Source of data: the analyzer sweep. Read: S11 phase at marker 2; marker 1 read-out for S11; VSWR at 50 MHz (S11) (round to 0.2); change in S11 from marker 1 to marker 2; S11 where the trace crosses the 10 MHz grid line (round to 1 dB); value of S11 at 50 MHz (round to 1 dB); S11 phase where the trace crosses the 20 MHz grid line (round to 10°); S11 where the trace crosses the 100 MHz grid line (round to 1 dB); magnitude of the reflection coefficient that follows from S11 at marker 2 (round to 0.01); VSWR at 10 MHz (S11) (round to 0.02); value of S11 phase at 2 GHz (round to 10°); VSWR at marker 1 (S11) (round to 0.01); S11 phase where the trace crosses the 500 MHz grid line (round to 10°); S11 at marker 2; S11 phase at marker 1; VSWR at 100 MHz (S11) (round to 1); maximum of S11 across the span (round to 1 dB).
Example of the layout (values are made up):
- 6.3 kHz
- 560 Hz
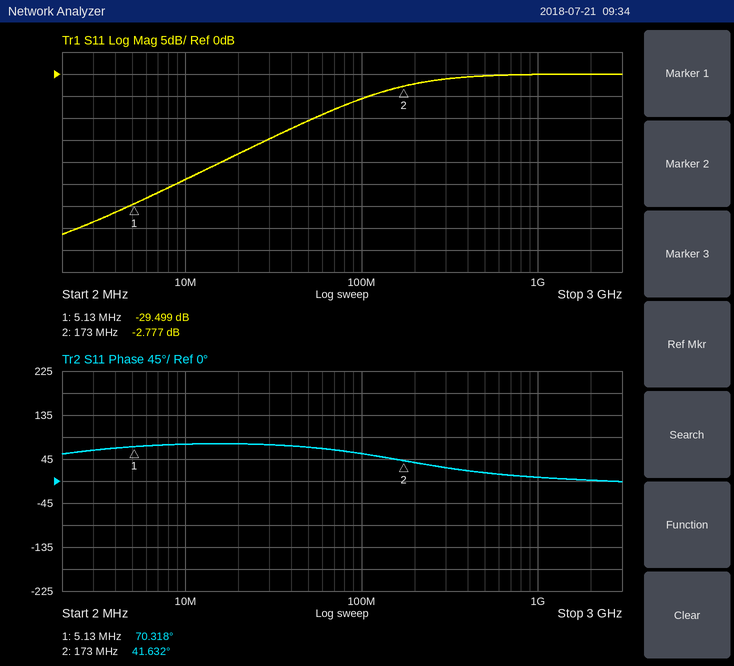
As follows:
- 41.632°
- -29.499 dB
- 1.8
- 26.722 dB
- -24 dB
- -11 dB
- 80°
- -6 dB
- 0.73
- 1.14
- 0°
- 1.07
- 20°
- -2.777 dB
- 70.318°
- 3
- 0 dB
